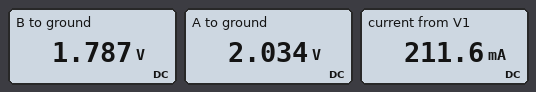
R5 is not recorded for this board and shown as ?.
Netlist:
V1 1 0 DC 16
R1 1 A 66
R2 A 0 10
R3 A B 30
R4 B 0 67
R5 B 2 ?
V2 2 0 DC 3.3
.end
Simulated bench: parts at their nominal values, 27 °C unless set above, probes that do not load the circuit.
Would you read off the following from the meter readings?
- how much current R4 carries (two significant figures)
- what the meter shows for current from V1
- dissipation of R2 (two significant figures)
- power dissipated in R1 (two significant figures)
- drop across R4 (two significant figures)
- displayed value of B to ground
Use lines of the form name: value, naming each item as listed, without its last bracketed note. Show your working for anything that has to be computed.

how much current R4 carries: (1.787 V) / 67 Ω = 27 mA
what the meter shows for current from V1: 211.6 mA
dissipation of R2: (2.034 V)^2 / 10 Ω = 410 mW
power dissipated in R1: (16 V - 2.034 V)^2 / 66 Ω = 3.0 W
drop across R4: 1.787 V = 1.8 V
displayed value of B to ground: 1.787 V
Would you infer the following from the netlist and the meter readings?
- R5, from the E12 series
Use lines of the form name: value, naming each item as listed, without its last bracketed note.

R5, from the E12 series: 82 Ω
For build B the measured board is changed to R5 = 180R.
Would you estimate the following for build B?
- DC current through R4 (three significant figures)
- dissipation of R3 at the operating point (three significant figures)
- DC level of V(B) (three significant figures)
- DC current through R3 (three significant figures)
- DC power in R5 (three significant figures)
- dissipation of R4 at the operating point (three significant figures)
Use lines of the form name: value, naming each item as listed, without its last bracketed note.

DC current through R4: 23.4 mA
dissipation of R3 at the operating point: 5.74 mW
DC level of V(B): 1.57 V
DC current through R3: 13.8 mA
DC power in R5: 16.6 mW
dissipation of R4 at the operating point: 36.8 mW
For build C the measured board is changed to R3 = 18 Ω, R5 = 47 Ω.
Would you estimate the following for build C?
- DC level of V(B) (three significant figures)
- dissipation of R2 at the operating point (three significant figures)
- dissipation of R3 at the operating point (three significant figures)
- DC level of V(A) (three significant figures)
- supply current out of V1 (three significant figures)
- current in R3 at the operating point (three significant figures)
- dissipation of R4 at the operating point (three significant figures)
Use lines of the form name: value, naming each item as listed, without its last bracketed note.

DC level of V(B): 2.02 V
dissipation of R2 at the operating point: 432 mW
dissipation of R3 at the operating point: 168 µW
DC level of V(A): 2.08 V
supply current out of V1: 211 mA
current in R3 at the operating point: 3.05 mA
dissipation of R4 at the operating point: 61.1 mW
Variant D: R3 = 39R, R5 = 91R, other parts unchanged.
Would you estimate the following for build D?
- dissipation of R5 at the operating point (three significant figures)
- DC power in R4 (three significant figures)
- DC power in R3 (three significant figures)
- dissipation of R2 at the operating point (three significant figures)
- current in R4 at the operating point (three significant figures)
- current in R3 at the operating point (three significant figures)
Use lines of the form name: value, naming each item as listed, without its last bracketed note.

dissipation of R5 at the operating point: 27.6 mW
DC power in R4: 43.9 mW
DC power in R3: 2.61 mW
dissipation of R2 at the operating point: 414 mW
current in R4 at the operating point: 25.6 mA
current in R3 at the operating point: 8.18 mA
